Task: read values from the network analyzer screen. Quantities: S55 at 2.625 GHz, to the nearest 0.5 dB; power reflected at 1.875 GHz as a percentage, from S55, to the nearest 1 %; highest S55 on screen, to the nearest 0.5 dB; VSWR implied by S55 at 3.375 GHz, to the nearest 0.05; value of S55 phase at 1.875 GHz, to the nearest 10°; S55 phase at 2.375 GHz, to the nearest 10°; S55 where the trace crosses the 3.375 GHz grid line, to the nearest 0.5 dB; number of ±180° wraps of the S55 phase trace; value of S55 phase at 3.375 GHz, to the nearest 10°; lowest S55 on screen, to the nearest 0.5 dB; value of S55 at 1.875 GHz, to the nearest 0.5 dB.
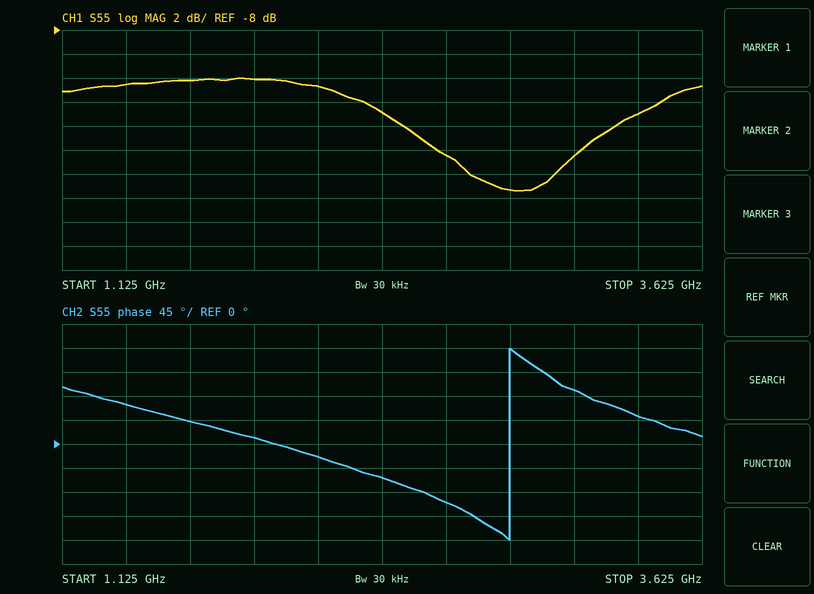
-18.5 dB
6 %
-12.0 dB
1.45
10°
-60°
-15.0 dB
1
50°
-21.5 dB
-12.0 dB
